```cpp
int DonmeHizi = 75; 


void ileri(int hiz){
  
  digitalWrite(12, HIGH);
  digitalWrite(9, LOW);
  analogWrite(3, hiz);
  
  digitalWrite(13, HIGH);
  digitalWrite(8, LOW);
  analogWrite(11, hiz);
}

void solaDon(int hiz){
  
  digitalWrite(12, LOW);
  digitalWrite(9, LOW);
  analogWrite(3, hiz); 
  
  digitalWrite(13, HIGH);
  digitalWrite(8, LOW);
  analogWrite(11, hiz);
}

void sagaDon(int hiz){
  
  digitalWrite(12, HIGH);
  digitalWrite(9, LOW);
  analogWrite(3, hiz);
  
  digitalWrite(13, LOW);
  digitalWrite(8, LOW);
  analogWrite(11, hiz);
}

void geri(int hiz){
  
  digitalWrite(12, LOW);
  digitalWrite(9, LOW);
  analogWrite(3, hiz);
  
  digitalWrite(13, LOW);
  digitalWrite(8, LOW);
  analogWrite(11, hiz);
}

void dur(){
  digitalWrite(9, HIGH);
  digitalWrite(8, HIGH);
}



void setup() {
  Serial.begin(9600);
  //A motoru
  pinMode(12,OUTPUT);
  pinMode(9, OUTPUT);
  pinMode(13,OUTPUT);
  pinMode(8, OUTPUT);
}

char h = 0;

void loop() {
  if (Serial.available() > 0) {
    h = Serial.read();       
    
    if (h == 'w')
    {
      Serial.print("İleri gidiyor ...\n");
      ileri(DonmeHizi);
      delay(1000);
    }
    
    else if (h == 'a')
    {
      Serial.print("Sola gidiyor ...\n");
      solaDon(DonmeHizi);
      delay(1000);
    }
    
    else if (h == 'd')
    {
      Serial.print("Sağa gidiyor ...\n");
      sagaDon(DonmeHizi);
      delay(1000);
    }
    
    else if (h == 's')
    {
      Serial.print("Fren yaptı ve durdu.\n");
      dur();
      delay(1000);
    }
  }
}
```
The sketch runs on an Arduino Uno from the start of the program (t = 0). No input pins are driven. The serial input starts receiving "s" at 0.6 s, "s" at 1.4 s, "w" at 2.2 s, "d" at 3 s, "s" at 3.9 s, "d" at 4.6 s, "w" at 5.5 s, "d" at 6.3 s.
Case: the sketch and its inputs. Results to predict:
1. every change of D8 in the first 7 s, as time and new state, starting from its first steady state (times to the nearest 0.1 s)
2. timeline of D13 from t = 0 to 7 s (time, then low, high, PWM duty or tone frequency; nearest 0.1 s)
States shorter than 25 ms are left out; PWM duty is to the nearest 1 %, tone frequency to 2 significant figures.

0 s low; 0.6 s high; 2.6 s low; 4.6 s high; 5.6 s low
0 s low; 2.6 s high; 3.6 s low; 6.6 s high
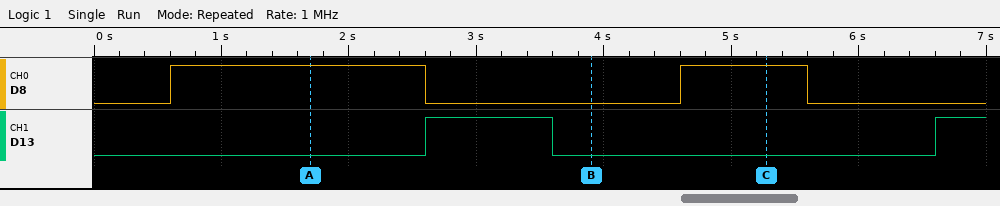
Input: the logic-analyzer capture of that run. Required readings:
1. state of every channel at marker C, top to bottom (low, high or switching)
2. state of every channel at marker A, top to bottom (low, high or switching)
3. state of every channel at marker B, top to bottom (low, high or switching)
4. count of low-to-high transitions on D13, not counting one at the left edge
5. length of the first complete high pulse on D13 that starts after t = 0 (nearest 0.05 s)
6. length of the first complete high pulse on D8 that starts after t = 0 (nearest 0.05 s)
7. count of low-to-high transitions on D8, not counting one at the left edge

D8 high, D13 low
D8 high, D13 low
D8 low, D13 low
2
1.00 s
2.00 s
2
